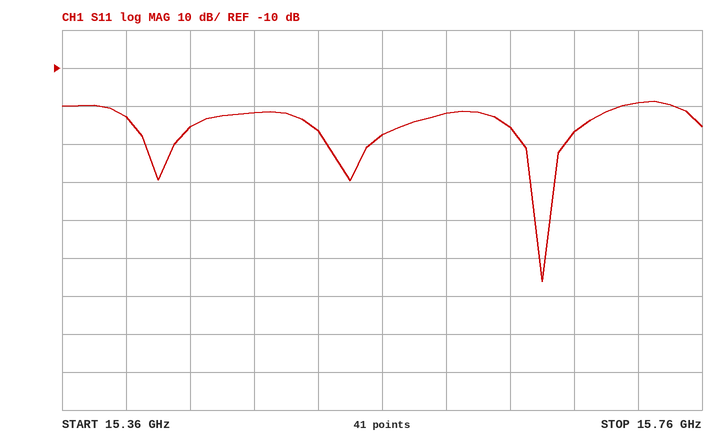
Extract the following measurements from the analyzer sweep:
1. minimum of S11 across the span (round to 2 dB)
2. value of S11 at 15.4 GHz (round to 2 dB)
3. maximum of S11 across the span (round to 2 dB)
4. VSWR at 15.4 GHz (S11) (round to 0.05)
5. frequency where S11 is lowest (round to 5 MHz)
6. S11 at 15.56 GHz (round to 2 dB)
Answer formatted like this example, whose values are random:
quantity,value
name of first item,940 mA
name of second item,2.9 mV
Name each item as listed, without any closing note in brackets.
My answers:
quantity,value
minimum of S11 across the span,-66 dB
value of S11 at 15.4 GHz,-22 dB
maximum of S11 across the span,-18 dB
VSWR at 15.4 GHz (S11),1.15
frequency where S11 is lowest,15.660 GHz
S11 at 15.56 GHz,-28 dB
